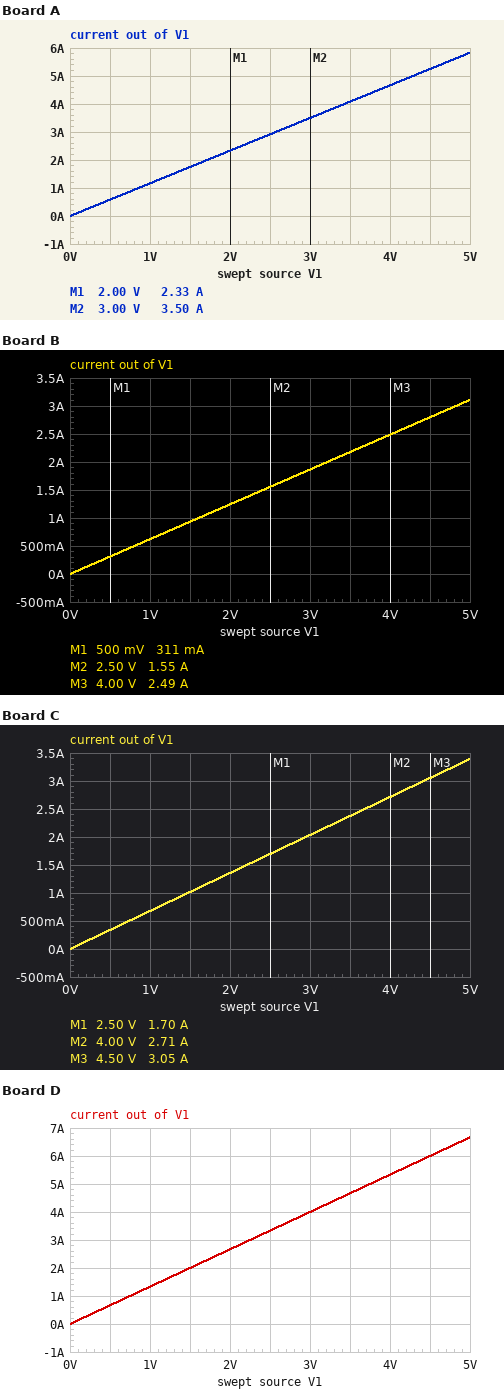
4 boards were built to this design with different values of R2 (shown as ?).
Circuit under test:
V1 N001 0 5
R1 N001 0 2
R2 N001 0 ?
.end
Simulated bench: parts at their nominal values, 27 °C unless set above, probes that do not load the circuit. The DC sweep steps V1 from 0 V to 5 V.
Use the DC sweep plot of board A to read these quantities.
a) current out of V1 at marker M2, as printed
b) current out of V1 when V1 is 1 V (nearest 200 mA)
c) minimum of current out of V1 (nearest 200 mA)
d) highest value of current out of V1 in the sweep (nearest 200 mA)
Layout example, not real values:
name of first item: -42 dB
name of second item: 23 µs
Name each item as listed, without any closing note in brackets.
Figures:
current out of V1 at marker M2, as printed: 3.50 A
current out of V1 when V1 is 1 V: 1.2 A
minimum of current out of V1: 0 A
highest value of current out of V1 in the sweep: 5.8 A
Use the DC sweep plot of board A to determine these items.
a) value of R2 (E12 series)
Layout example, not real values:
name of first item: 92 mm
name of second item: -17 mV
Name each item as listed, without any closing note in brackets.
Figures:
value of R2: 1.5 Ω
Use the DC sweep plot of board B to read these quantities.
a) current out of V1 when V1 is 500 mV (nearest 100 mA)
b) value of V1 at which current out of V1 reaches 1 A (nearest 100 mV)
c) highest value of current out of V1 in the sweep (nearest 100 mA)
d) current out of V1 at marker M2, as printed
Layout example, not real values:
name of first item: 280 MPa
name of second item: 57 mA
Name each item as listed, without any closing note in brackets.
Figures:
current out of V1 when V1 is 500 mV: 300 mA
value of V1 at which current out of V1 reaches 1 A: 1.6 V
highest value of current out of V1 in the sweep: 3.1 A
current out of V1 at marker M2, as printed: 1.55 A
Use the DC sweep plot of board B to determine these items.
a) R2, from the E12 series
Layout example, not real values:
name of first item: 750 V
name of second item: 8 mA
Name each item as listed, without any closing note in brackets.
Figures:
R2, from the E12 series: 8.2 Ω
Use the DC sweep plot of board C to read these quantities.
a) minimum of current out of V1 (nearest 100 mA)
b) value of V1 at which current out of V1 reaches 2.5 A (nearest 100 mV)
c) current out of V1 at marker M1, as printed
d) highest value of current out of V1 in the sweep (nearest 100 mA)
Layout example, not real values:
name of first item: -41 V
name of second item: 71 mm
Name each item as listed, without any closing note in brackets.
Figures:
minimum of current out of V1: 0 A
value of V1 at which current out of V1 reaches 2.5 A: 3.7 V
current out of V1 at marker M1, as printed: 1.70 A
highest value of current out of V1 in the sweep: 3.4 A
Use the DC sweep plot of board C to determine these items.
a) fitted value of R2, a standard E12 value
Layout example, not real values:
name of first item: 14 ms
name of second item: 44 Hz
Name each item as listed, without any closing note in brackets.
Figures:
fitted value of R2, a standard E12 value: 5.6 Ω
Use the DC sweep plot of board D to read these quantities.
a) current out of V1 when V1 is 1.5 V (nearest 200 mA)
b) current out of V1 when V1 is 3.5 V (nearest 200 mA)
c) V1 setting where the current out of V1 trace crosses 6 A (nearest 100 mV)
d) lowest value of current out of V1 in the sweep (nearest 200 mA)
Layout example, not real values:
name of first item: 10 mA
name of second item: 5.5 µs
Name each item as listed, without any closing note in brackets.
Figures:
current out of V1 when V1 is 1.5 V: 2.0 A
current out of V1 when V1 is 3.5 V: 4.6 A
V1 setting where the current out of V1 trace crosses 6 A: 4.5 V
lowest value of current out of V1 in the sweep: 0 A
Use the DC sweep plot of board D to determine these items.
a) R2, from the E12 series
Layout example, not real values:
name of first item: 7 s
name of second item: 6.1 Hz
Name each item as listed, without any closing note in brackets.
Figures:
R2, from the E12 series: 1.2 Ω
